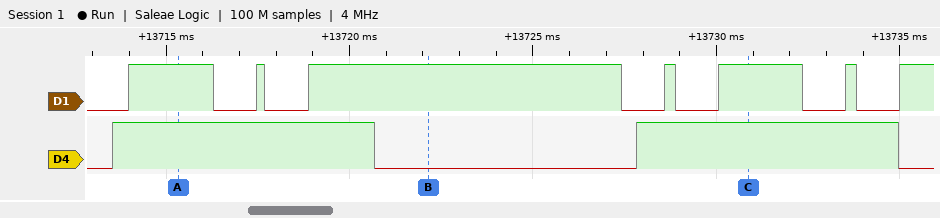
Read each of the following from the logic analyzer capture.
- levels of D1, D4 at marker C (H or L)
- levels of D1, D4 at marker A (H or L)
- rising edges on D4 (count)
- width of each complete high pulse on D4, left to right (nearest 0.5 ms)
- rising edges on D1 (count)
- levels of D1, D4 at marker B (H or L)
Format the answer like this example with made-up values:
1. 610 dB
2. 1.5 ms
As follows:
1. D1=H, D4=H
2. D1=H, D4=H
3. 2
4. 7 ms, 7 ms
5. 7
6. D1=H, D4=L
